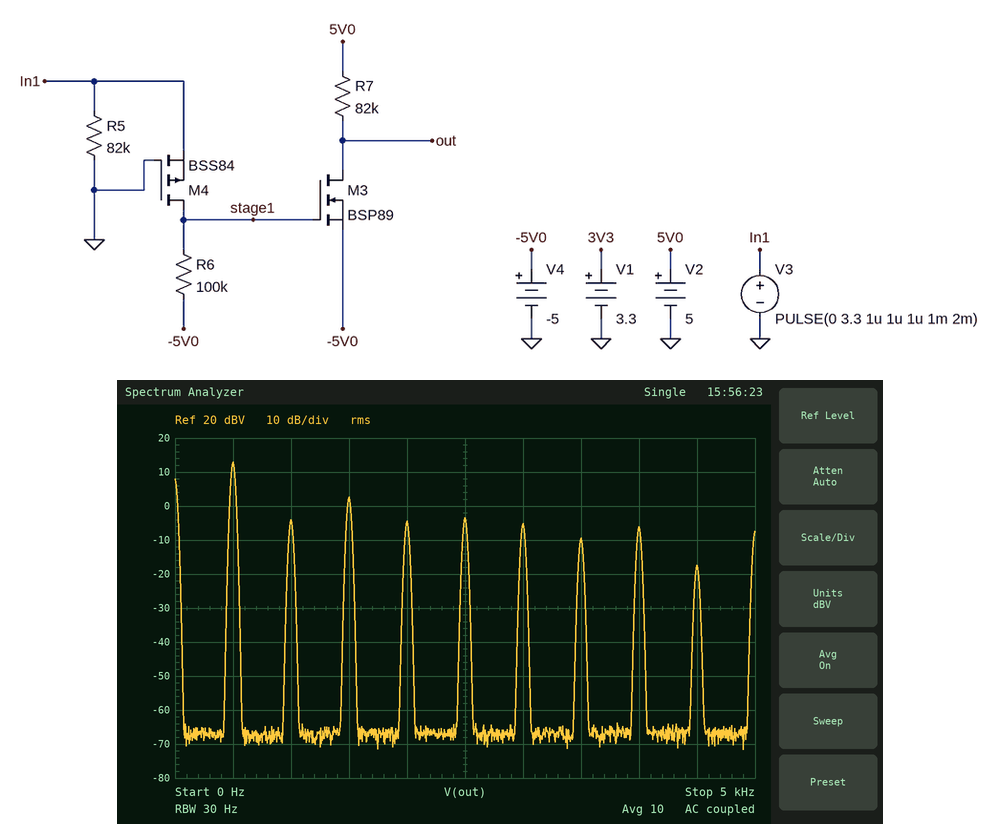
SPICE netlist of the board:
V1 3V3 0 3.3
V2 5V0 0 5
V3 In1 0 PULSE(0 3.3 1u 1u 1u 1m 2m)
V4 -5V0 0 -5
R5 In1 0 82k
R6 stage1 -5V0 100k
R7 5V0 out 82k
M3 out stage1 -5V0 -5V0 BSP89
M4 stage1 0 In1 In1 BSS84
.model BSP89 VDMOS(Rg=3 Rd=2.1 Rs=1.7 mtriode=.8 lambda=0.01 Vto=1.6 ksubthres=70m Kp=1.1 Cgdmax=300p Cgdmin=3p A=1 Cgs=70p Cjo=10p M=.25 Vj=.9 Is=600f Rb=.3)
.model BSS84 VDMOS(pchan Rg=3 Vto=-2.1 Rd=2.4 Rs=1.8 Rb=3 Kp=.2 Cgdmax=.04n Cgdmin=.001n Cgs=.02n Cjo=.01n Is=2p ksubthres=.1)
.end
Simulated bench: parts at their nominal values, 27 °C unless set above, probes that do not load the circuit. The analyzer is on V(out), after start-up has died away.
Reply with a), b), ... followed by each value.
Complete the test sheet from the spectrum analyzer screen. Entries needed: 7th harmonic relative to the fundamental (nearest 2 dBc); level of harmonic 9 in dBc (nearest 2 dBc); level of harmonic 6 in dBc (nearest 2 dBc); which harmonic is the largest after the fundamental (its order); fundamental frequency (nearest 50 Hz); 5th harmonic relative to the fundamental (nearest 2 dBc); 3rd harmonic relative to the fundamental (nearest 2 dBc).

a) -22 dBc
b) -30 dBc
c) -18 dBc
d) 3
e) 500 Hz
f) -16 dBc
g) -10 dBc
